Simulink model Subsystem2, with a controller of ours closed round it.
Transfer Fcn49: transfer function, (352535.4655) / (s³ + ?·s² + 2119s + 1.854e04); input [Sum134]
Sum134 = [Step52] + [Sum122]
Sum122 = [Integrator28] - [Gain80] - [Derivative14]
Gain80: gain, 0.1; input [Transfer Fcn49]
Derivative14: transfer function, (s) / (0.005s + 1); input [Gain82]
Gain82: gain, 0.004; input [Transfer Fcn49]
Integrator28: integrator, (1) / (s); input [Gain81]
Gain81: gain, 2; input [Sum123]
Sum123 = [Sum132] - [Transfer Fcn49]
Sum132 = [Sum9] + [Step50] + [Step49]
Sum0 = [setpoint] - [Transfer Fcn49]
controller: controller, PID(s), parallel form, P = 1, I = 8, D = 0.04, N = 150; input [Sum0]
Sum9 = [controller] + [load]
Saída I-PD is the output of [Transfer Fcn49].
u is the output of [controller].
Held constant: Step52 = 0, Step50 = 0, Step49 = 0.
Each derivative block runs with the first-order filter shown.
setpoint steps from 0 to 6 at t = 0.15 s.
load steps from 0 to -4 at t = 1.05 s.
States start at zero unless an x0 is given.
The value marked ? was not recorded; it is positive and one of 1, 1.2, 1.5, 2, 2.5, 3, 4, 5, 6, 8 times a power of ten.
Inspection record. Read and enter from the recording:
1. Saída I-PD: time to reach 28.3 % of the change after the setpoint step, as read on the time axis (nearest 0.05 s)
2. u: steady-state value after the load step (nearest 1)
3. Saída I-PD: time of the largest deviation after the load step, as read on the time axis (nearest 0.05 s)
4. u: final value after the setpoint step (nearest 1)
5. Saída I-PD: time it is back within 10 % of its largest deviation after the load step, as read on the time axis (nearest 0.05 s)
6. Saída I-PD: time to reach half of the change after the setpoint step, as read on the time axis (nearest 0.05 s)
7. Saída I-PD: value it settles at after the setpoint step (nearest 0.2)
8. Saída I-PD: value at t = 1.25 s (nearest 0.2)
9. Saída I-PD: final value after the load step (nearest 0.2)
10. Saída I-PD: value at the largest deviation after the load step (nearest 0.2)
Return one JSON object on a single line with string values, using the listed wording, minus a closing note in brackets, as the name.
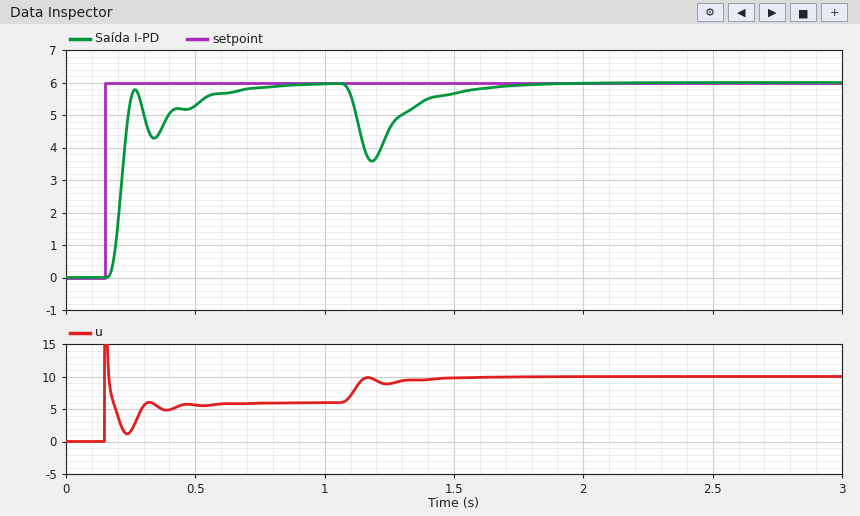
{"Saída I-PD: time to reach 28.3 % of the change after the setpoint step, as read on the time axis": "0.20 s", "u: steady-state value after the load step": "10", "Saída I-PD: time of the largest deviation after the load step, as read on the time axis": "1.20 s", "u: final value after the setpoint step": "6", "Saída I-PD: time it is back within 10 % of its largest deviation after the load step, as read on the time axis": "1.55 s", "Saída I-PD: time to reach half of the change after the setpoint step, as read on the time axis": "0.20 s", "Saída I-PD: value it settles at after the setpoint step": "6.0", "Saída I-PD: value at t = 1.25 s": "4.6", "Saída I-PD: final value after the load step": "6.0", "Saída I-PD: value at the largest deviation after the load step": "3.6"}
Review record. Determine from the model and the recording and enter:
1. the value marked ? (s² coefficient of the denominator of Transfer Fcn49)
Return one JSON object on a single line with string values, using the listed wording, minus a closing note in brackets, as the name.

{"the value marked ?": "60"}
